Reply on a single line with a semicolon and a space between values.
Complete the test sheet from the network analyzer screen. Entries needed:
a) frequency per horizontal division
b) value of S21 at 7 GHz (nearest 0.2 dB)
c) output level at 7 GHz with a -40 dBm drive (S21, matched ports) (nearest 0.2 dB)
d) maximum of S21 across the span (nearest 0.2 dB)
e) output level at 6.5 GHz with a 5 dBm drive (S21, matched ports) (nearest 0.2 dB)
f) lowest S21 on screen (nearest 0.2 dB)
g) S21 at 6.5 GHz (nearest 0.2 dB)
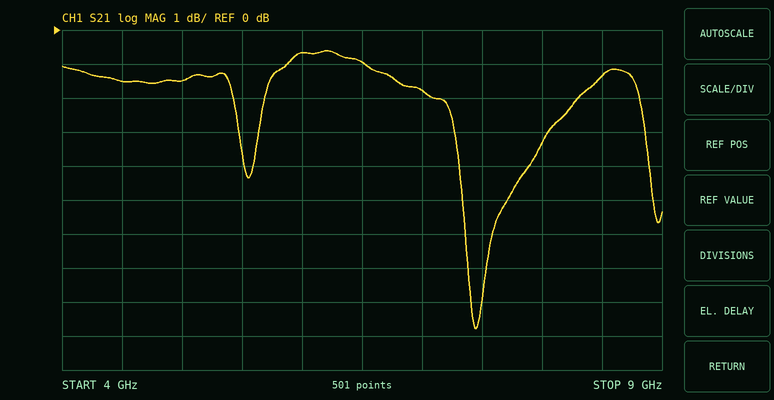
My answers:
500 MHz; -1.8 dB; -41.8 dBm; -0.6 dB; 4.0 dBm; -8.8 dB; -1.0 dB
